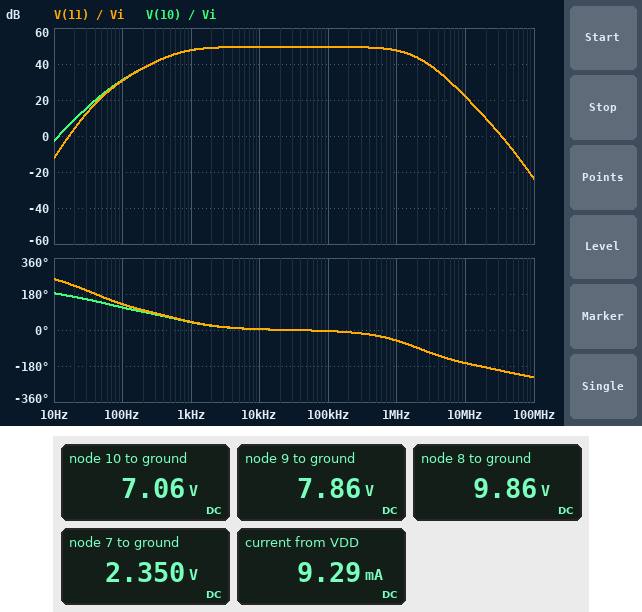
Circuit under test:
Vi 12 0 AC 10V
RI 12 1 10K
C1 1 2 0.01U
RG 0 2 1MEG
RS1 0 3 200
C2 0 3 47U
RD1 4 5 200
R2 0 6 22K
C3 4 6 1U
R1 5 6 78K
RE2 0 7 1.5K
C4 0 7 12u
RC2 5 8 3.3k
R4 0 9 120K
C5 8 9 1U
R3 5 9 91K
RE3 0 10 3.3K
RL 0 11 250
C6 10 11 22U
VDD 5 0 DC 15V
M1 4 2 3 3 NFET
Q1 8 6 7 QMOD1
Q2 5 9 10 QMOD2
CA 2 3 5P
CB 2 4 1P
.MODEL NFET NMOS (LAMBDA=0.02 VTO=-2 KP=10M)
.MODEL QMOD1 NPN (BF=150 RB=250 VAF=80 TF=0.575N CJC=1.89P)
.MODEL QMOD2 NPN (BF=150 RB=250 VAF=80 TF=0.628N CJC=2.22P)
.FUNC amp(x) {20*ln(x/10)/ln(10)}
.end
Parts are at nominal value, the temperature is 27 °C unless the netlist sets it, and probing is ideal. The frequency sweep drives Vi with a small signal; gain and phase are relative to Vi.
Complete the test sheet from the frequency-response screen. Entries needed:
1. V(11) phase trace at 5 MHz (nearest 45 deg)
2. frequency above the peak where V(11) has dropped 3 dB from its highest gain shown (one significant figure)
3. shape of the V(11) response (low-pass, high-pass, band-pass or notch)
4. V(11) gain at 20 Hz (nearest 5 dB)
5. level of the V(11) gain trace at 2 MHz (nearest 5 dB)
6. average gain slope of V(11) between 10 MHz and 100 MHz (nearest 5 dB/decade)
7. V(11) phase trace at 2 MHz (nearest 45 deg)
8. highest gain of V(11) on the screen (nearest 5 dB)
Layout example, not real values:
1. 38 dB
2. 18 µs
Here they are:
1. -135 deg
2. 1 MHz
3. band-pass
4. 5 dB
5. 45 dB
6. -45 dB/decade
7. -90 deg
8. 50 dB
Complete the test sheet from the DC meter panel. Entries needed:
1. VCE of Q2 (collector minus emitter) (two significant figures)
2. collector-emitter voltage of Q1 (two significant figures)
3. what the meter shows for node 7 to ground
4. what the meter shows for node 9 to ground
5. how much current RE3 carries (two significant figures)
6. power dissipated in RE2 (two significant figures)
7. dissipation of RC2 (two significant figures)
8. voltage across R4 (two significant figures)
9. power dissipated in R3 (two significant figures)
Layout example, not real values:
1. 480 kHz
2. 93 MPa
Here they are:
1. 7.9 V
2. 7.5 V
3. 2.350 V
4. 7.86 V
5. 2.1 mA
6. 3.7 mW
7. 8.0 mW
8. 7.9 V
9. 560 µW
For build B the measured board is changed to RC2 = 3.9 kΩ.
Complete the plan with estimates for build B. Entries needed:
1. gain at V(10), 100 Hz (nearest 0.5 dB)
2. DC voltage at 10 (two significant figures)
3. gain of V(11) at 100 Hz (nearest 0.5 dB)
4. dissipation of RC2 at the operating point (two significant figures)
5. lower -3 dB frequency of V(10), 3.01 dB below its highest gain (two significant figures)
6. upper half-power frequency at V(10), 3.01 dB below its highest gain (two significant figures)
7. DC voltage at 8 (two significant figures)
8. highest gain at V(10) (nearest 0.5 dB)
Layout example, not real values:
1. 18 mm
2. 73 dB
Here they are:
1. 32.5 dB
2. 7.1 V
3. 32.0 dB
4. 9.4 mW
5. 710 Hz
6. 1.2 MHz
7. 8.9 V
8. 50.5 dB
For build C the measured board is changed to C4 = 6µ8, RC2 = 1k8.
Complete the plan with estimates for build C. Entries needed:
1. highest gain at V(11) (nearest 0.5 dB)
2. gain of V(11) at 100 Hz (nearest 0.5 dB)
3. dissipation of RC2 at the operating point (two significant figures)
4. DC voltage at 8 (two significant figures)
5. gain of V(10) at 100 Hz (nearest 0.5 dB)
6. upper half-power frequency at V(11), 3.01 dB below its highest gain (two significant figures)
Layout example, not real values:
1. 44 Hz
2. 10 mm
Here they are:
1. 45.0 dB
2. 21.5 dB
3. 4.4 mW
4. 12 V
5. 22.0 dB
6. 1.5 MHz
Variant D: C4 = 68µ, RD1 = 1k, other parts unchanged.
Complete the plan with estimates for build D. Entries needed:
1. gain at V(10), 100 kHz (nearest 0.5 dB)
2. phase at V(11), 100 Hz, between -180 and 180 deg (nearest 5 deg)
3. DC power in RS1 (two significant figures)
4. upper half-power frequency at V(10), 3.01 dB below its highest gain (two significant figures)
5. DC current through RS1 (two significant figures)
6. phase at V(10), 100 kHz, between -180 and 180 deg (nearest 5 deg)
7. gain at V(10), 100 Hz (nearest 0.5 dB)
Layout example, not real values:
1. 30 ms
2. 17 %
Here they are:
1. 60.5 dB
2. 100 deg
3. 5.5 mW
4. 660 kHz
5. 5.3 mA
6. -10 deg
7. 55.0 dB
